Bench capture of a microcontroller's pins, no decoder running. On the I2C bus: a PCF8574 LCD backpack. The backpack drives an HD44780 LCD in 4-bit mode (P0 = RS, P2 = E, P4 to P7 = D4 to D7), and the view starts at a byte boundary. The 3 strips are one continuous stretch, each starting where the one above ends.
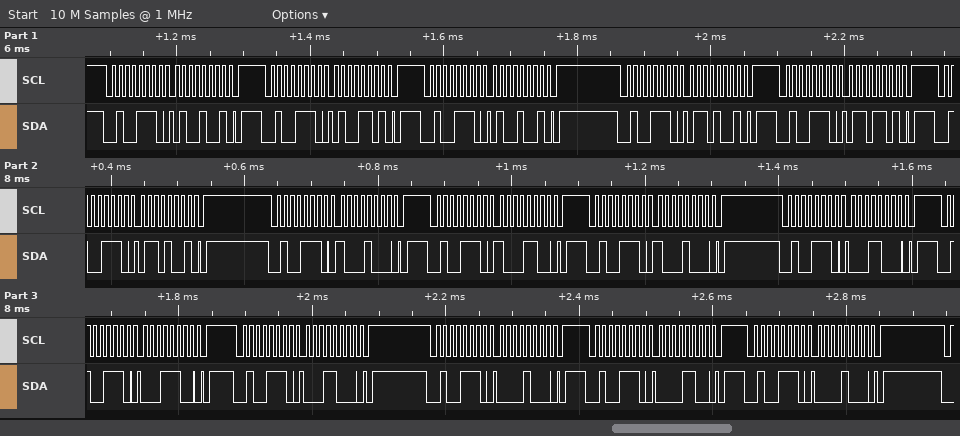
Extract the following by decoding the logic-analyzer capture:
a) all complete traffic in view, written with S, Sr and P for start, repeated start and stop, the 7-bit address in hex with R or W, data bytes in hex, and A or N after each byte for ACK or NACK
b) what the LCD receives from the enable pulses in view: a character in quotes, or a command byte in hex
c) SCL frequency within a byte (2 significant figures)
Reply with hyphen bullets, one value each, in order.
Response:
- S 27W A 49 A P S 27W A 4D A P S 27W A 49 A P S 27W A 69 A P S 27W A 6D A P S 27W A 69 A P S 27W A 88 A P S 27W A 8C A P S 27W A 88 A P S 27W A 18 A P S 27W A 1C A P S 27W A 18 A P S 27W A 08 A P S 27W A 0C A P S 27W A 08 A P
- 'F' 0x81
- 100 kHz
